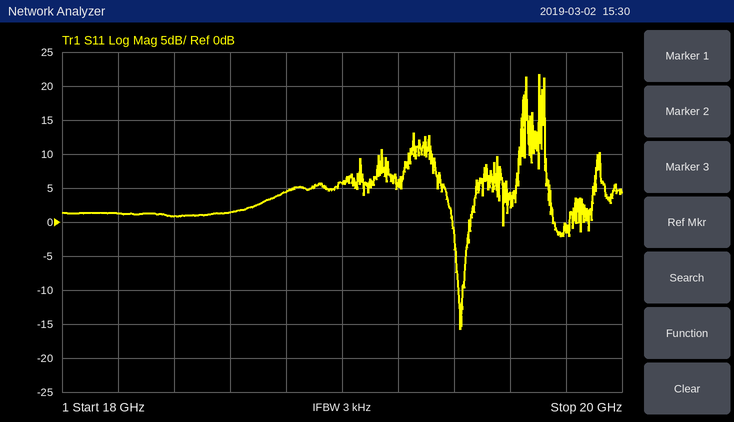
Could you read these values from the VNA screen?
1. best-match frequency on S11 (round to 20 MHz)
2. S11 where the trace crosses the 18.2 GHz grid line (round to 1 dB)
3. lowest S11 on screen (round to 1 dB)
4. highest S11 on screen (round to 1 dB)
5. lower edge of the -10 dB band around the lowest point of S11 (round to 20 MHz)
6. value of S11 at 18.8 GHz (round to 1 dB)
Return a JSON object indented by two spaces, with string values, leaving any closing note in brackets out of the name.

{
  "best-match frequency on S11": "19.42 GHz",
  "S11 where the trace crosses the 18.2 GHz grid line": "1 dB",
  "lowest S11 on screen": "-16 dB",
  "highest S11 on screen": "22 dB",
  "lower edge of the -10 dB band around the lowest point of S11": "19.42 GHz",
  "value of S11 at 18.8 GHz": "4 dB"
}
